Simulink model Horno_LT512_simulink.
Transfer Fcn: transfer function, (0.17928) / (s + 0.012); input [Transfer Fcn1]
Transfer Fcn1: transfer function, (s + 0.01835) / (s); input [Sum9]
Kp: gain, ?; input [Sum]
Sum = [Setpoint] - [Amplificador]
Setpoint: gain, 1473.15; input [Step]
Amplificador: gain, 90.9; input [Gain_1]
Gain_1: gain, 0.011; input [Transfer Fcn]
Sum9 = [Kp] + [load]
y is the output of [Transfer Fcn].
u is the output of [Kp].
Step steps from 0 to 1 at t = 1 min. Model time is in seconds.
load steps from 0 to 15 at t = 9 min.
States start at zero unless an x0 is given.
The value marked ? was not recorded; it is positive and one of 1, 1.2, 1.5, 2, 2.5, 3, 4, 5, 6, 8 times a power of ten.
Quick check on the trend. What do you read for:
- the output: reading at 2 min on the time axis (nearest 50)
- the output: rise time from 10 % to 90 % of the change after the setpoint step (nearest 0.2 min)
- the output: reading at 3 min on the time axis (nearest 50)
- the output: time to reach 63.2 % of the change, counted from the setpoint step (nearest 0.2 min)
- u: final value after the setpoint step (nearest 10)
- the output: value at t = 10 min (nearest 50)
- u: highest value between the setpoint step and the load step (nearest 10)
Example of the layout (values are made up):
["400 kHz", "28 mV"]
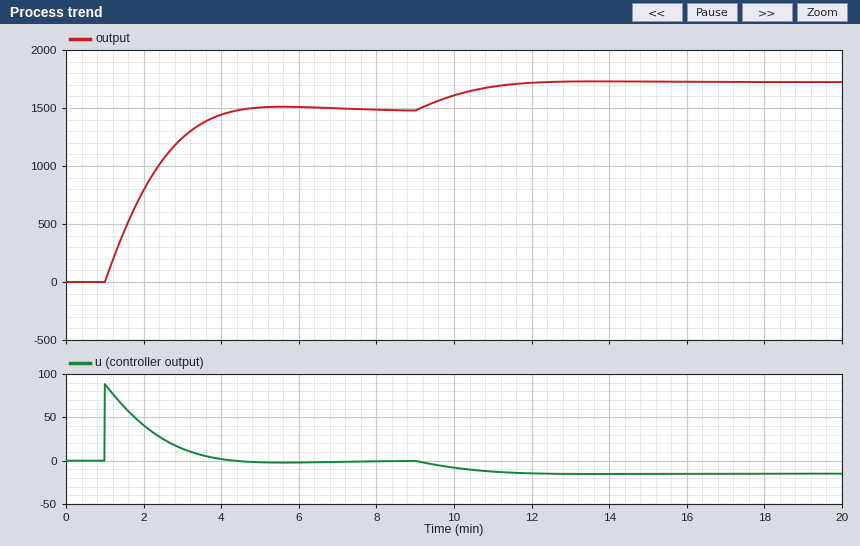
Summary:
["800", "2.2 min", "1250", "1.2 min", "0", "1600", "90"]
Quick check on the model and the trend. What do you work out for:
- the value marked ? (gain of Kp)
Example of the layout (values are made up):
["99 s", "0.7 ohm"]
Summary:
["0.06"]
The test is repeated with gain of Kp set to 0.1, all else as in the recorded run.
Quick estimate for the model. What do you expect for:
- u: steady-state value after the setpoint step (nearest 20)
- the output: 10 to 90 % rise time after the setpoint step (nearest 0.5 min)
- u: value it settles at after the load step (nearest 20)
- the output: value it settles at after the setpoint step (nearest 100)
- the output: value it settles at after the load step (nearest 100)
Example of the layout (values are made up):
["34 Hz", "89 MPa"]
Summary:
["0", "1.5 min", "-20", "1500", "1600"]
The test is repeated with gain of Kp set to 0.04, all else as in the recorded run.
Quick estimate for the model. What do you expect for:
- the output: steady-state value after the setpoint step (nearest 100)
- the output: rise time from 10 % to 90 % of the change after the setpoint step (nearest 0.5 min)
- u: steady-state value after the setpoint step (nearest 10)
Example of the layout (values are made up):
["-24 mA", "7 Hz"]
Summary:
["1500", "3.0 min", "0"]
